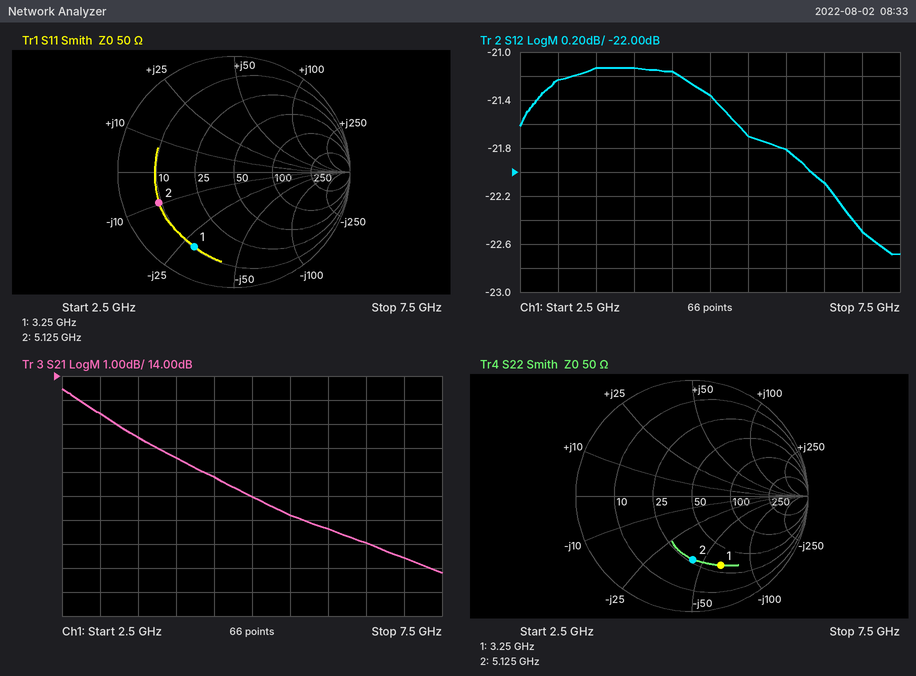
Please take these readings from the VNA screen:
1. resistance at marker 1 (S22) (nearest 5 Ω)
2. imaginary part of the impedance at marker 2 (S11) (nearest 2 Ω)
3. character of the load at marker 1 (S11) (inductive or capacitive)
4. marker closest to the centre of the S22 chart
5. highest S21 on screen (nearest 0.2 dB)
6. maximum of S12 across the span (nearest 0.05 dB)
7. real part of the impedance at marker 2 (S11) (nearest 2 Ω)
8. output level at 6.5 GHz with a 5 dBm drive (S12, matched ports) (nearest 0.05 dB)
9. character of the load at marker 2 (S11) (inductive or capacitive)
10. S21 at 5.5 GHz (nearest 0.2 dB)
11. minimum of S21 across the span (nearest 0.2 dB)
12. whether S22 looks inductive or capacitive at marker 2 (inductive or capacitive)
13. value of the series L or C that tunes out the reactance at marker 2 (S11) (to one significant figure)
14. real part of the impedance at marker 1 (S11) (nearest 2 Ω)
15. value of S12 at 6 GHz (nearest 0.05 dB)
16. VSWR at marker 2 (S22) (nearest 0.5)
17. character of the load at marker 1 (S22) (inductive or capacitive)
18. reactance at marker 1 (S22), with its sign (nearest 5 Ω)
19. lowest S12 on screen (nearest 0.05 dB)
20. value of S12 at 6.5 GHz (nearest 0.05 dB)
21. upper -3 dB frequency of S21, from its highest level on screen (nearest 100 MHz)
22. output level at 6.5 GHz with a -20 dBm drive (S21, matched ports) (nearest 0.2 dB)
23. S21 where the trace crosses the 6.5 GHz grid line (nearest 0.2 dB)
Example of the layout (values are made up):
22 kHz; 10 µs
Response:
30 Ω; -10 Ω; capacitive; marker 2; 13.4 dB; -21.15 dB; 10 Ω; -17.10 dBm; capacitive; 8.2 dB; 5.8 dB; capacitive; 300 pH; 10 Ω; -21.80 dB; 3.5; capacitive; -65 Ω; -22.70 dB; -22.10 dB; 4.1 GHz; -13.0 dBm; 7.0 dB
